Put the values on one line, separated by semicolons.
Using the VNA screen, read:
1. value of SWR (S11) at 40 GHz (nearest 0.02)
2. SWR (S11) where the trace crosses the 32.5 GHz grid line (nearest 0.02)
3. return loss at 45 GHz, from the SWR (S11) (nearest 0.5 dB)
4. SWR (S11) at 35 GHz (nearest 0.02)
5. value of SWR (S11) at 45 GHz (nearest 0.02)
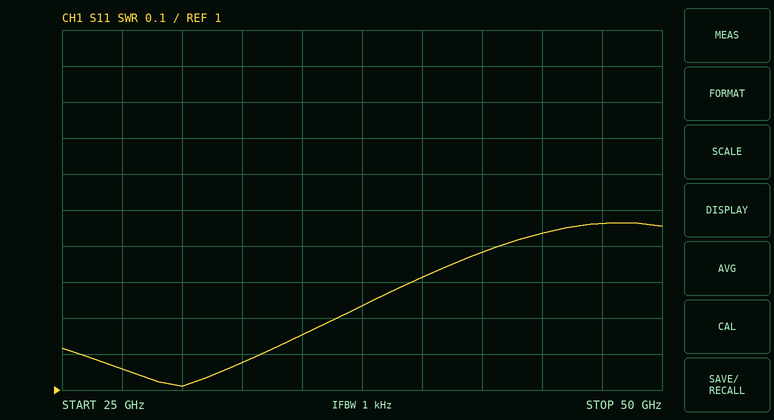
1.32; 1.08; 15.0 dB; 1.16; 1.44
